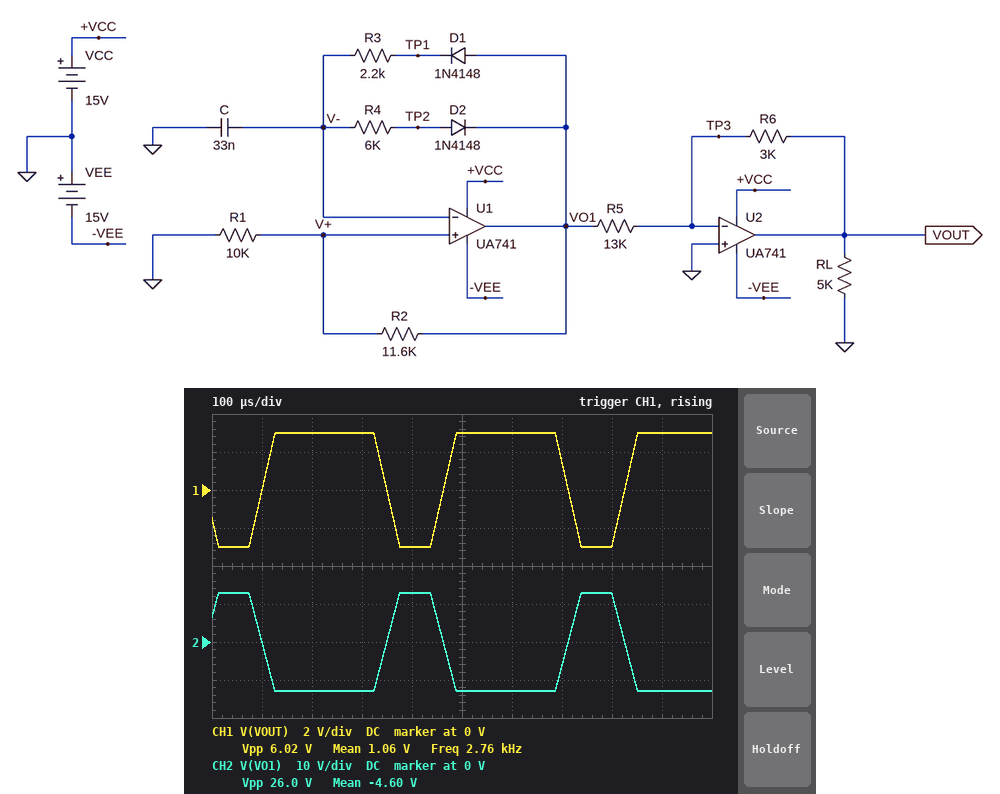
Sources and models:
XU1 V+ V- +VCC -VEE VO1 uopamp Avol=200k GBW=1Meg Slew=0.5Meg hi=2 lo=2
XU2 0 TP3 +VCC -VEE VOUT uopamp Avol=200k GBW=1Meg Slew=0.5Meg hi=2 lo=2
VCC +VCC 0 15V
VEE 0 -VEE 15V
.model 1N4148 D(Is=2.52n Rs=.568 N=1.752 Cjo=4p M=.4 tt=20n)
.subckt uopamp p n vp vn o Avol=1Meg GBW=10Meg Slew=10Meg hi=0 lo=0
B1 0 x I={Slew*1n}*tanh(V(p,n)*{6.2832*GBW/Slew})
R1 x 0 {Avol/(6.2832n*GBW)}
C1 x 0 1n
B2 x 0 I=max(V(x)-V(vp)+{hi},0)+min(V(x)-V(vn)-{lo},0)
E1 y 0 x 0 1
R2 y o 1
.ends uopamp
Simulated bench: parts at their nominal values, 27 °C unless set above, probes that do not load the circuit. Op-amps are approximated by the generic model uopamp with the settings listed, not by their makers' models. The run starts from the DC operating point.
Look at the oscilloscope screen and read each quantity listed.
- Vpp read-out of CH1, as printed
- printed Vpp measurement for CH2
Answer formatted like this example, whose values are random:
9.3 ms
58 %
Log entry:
6.02 V
26.0 V
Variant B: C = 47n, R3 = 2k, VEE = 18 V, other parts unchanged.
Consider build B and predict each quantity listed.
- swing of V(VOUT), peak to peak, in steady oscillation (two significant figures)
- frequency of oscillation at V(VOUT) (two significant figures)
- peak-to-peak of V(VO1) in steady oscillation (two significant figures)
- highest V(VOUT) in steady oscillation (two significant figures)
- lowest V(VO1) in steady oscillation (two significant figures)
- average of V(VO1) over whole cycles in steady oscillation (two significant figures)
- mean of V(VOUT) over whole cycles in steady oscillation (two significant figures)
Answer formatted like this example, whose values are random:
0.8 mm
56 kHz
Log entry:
6.7 V
2.1 kHz
29 V
3.7 V
-16 V
-6.9 V
1.6 V
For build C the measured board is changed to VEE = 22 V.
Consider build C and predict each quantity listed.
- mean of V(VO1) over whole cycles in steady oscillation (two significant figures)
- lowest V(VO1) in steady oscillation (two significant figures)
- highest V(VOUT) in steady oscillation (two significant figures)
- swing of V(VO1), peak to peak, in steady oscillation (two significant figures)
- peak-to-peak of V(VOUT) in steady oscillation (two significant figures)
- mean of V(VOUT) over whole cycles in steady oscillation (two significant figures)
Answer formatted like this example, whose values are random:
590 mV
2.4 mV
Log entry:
-7.6 V
-20 V
4.6 V
33 V
7.6 V
1.8 V
